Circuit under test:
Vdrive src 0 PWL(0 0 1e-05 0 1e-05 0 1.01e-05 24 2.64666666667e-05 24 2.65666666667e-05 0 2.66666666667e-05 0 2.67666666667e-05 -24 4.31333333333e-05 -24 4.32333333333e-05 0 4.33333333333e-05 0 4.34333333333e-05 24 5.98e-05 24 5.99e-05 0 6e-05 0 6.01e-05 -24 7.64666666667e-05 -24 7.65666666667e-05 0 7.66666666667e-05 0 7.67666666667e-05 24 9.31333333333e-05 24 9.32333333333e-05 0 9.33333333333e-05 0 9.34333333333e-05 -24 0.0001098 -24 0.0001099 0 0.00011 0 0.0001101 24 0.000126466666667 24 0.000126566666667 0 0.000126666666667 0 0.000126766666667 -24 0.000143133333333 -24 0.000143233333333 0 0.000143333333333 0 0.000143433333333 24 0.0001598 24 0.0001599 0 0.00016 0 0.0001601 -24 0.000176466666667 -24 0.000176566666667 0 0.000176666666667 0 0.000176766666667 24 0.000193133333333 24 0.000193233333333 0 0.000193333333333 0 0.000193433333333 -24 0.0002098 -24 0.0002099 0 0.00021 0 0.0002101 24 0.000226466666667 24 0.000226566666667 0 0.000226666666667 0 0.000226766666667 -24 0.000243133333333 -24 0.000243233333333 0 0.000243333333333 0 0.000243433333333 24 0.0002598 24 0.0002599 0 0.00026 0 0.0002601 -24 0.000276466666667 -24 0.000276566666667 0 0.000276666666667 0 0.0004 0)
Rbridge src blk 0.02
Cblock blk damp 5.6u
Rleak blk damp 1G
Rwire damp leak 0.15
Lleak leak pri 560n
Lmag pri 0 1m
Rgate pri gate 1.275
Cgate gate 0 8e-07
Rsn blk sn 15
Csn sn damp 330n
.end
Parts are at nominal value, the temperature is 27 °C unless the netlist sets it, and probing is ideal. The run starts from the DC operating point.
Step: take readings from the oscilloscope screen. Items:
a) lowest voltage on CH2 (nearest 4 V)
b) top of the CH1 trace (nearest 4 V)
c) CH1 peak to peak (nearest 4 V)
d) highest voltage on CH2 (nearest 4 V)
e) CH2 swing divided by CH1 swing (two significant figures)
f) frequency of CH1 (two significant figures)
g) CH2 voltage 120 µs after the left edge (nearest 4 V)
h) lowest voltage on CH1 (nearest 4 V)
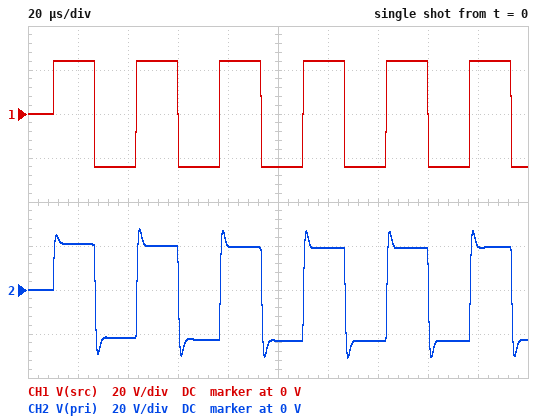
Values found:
-32 V
24 V
48 V
28 V
1.2
30 kHz
20 V
-24 V
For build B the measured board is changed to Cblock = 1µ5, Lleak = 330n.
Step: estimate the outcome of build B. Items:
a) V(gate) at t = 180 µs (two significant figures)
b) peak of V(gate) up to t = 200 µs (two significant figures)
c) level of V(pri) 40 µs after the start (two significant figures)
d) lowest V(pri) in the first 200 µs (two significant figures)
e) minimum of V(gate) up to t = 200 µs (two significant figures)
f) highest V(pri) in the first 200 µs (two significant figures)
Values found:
16 V
18 V
-18 V
-28 V
-19 V
26 V
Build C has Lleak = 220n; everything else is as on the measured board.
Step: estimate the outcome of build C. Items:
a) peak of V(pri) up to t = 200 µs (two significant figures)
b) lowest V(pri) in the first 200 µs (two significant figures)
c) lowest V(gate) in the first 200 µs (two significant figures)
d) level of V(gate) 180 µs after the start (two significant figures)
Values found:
24 V
-27 V
-23 V
18 V
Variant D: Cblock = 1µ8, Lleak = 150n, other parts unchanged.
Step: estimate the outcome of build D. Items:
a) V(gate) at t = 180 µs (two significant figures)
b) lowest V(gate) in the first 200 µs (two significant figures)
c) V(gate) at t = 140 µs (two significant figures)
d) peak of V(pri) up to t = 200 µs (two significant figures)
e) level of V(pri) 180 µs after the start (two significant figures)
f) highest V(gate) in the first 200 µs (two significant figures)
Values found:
16 V
-20 V
-19 V
25 V
17 V
18 V
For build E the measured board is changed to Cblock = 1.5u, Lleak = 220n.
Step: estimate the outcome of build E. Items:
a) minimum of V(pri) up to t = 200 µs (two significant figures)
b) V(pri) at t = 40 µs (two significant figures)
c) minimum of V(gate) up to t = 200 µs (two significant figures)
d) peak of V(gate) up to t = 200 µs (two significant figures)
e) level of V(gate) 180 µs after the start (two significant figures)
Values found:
-28 V
-18 V
-19 V
18 V
16 V
